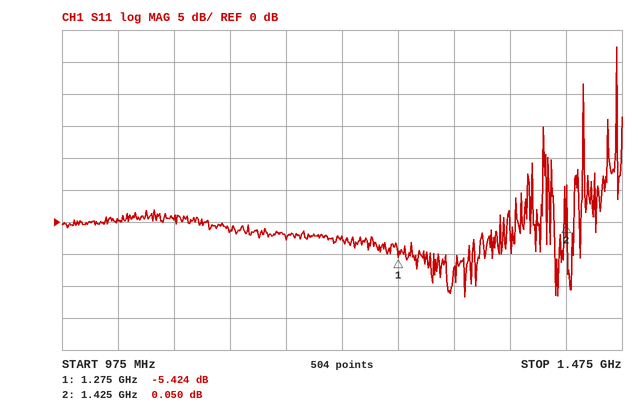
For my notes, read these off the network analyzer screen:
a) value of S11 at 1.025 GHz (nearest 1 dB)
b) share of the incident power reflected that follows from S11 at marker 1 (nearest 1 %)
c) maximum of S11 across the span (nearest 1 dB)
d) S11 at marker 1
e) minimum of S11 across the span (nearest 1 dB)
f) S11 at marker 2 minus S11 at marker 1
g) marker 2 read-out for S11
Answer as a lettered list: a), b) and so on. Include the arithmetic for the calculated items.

a) 0 dB
b) 10^(-5.424/10) ≈ 29 %
c) 27 dB
d) -5.424 dB
e) -12 dB
f) 0.05 − (-5.424) = 5.474 dB
g) 0.050 dB
